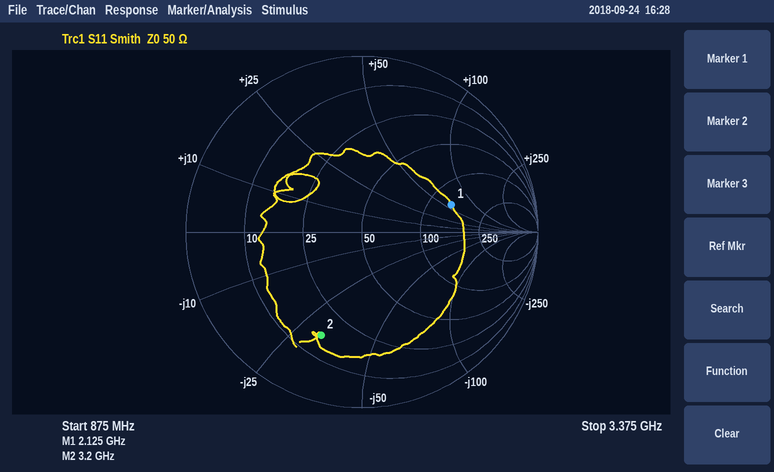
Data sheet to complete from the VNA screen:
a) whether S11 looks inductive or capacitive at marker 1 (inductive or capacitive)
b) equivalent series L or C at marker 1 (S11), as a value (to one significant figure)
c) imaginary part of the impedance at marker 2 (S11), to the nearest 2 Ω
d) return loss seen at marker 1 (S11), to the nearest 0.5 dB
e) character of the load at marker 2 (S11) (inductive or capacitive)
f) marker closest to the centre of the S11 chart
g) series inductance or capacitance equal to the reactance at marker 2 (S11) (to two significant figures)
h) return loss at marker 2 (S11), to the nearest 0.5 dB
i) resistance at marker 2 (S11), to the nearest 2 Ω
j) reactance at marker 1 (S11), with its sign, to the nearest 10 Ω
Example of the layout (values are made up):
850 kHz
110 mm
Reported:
inductive
4 nH
-32 Ω
5.5 dB
capacitive
marker 1
1.6 pF
4.0 dB
16 Ω
+60 Ω
